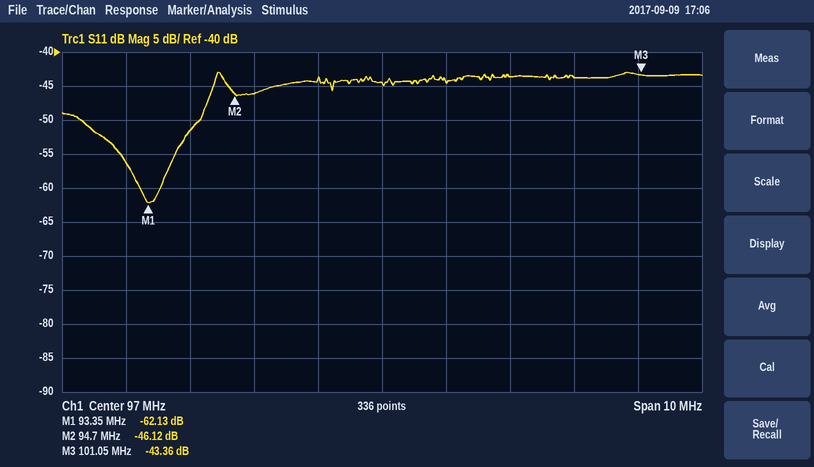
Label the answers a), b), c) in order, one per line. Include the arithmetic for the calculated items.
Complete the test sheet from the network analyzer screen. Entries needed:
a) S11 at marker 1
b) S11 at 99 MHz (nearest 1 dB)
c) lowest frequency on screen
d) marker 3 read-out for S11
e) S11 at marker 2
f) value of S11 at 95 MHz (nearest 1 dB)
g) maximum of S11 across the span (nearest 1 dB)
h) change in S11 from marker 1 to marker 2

a) -62.13 dB
b) -44 dB
c) 92 MHz
d) -43.36 dB
e) -46.12 dB
f) -46 dB
g) -43 dB
h) -46.12 − (-62.13) = 16.01 dB
